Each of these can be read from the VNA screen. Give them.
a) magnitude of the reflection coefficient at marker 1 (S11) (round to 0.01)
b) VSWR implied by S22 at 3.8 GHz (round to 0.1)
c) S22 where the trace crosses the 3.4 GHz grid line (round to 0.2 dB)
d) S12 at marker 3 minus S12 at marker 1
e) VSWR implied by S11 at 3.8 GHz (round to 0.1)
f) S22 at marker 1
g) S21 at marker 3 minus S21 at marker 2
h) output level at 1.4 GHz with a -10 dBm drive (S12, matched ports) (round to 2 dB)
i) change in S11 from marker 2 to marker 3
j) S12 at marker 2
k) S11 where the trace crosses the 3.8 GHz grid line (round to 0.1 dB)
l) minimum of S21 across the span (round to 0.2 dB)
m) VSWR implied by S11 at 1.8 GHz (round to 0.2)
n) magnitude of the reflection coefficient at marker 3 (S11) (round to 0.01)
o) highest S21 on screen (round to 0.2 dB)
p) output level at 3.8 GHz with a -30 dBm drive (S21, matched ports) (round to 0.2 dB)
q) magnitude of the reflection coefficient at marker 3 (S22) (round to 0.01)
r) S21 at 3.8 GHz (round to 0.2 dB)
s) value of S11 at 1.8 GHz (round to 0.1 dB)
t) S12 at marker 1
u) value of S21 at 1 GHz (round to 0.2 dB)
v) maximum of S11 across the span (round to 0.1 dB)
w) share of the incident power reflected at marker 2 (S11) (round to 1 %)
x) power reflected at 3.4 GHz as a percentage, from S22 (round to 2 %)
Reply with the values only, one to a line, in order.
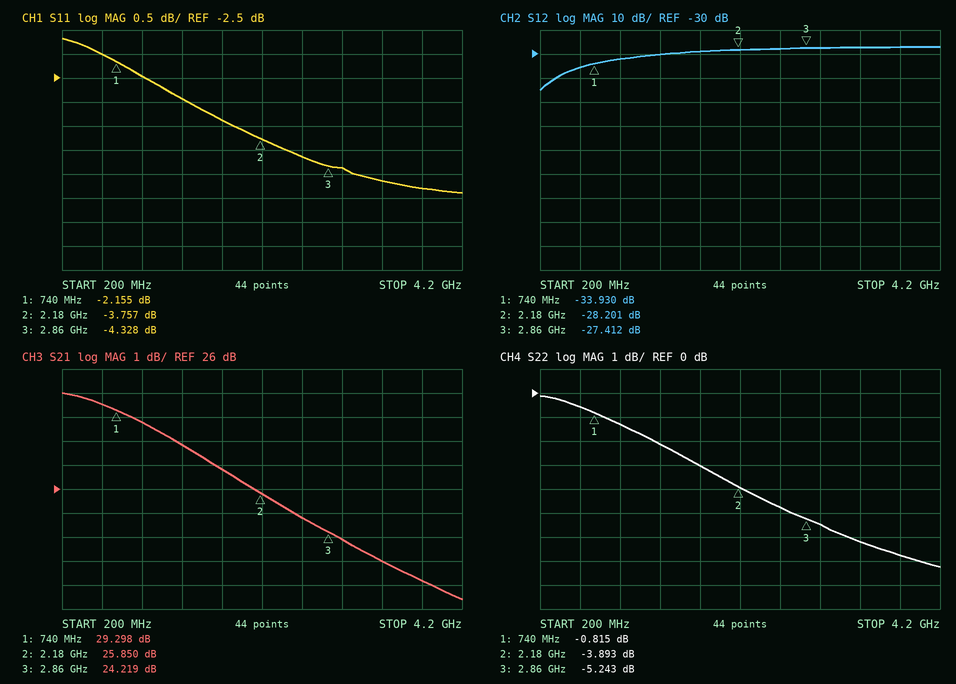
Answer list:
0.78
2.7
-6.2 dB
6.518 dB
3.7
-0.815 dB
-1.631 dB
-40 dBm
-0.571 dB
-28.201 dB
-4.8 dB
21.4 dB
5.2
0.61
30.0 dB
-7.8 dBm
0.55
22.2 dB
-3.4 dB
-33.930 dB
28.8 dB
-1.7 dB
42 %
24 %
